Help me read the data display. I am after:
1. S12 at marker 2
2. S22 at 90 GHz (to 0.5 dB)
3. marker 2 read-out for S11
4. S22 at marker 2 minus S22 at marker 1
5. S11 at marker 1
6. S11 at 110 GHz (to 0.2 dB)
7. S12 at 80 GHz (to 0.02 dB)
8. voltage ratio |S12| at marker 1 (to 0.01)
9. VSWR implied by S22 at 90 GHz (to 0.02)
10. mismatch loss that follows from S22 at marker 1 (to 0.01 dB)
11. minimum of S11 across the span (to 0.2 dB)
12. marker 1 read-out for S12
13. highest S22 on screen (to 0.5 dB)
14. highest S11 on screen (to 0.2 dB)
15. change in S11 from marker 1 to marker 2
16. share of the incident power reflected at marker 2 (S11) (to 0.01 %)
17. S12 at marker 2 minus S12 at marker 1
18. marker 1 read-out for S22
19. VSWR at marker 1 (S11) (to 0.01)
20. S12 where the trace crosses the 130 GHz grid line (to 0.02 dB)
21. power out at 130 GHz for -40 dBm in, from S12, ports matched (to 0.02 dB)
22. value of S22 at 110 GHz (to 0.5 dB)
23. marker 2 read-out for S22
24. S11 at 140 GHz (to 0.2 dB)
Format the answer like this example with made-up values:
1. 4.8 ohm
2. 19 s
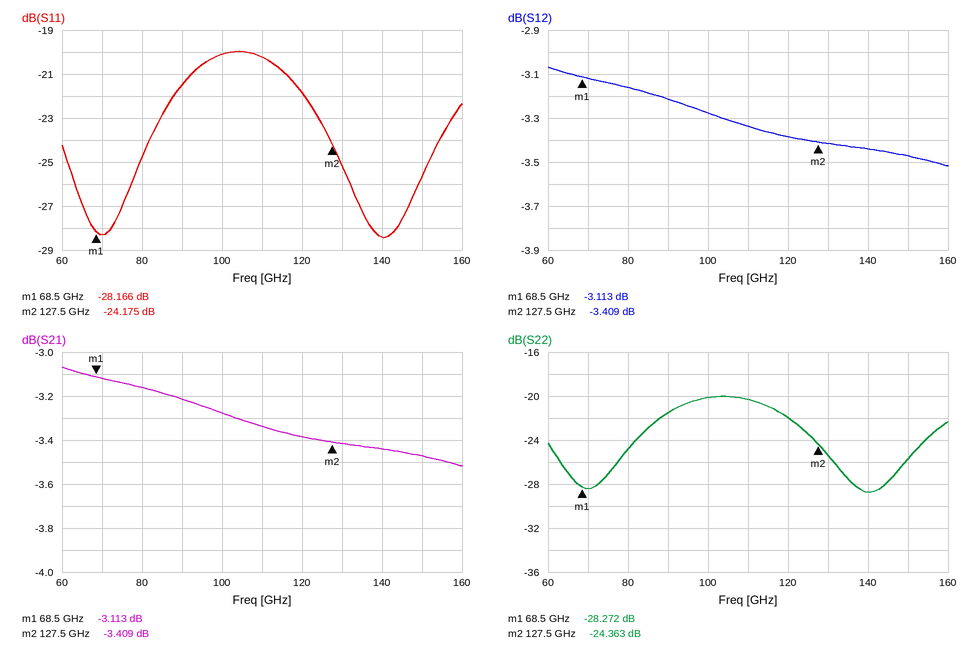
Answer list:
1. -3.409 dB
2. -21.5 dB
3. -24.175 dB
4. 3.909 dB
5. -28.166 dB
6. -20.2 dB
7. -3.16 dB
8. 0.70
9. 1.18
10. 0.01 dB
11. -28.4 dB
12. -3.113 dB
13. -20.0 dB
14. -20.0 dB
15. 3.991 dB
16. 0.38 %
17. -0.296 dB
18. -28.272 dB
19. 1.08
20. -3.42 dB
21. -43.42 dBm
22. -20.5 dB
23. -24.363 dB
24. -28.4 dB
